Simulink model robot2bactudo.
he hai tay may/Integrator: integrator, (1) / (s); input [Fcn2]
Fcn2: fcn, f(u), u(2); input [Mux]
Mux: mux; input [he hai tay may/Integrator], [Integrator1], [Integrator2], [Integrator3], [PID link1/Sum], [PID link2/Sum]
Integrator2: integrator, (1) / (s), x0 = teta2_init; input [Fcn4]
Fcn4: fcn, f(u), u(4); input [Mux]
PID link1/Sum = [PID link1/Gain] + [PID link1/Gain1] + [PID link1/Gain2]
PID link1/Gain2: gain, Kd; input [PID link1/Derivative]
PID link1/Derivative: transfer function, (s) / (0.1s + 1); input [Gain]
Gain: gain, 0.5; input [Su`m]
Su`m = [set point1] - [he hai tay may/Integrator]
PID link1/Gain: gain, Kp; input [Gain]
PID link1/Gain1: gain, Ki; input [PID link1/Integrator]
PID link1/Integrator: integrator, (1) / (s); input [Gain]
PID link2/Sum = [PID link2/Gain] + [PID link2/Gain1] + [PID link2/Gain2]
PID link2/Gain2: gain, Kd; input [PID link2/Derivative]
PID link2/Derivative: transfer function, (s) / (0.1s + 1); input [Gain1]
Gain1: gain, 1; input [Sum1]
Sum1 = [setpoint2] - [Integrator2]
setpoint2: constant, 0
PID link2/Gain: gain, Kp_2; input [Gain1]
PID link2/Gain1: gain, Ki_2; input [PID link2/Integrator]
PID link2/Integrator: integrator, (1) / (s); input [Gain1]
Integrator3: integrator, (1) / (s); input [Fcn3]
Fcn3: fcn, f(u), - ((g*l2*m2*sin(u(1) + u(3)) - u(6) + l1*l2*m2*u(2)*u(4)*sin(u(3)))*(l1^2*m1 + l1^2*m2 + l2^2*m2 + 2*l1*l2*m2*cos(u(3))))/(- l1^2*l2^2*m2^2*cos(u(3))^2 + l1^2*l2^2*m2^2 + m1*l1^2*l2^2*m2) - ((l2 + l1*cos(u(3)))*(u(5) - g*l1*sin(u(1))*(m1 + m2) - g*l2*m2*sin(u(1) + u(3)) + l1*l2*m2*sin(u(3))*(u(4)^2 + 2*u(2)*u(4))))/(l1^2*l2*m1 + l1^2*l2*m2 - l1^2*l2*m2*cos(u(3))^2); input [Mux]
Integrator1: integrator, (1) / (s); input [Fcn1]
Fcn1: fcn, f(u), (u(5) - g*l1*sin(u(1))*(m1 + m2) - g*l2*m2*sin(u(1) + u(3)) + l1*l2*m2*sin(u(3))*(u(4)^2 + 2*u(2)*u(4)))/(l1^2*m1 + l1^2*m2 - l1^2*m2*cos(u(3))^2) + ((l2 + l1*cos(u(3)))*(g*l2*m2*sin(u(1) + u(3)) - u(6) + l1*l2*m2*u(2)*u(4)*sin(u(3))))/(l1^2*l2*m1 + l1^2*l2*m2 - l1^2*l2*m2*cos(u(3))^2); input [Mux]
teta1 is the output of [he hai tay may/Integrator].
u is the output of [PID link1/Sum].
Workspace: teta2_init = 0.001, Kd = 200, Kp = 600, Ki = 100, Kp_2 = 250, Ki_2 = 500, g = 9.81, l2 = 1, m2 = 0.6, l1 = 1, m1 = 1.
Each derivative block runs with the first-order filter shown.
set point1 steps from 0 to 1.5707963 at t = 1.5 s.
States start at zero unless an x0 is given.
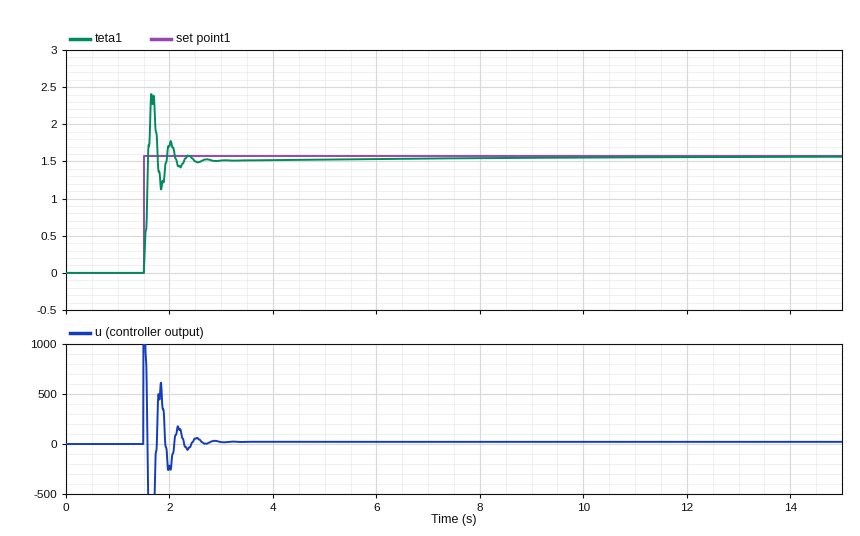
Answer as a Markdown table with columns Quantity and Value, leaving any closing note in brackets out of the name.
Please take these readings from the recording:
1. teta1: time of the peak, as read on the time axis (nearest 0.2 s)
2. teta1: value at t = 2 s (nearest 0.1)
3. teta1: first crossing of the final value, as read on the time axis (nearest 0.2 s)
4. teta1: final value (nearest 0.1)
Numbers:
| Quantity | Value |
|---|---|
| teta1: time of the peak, as read on the time axis | 1.6 s |
| teta1: value at t = 2 s | 1.7 |
| teta1: first crossing of the final value, as read on the time axis | 1.6 s |
| teta1: final value | 1.6 |
